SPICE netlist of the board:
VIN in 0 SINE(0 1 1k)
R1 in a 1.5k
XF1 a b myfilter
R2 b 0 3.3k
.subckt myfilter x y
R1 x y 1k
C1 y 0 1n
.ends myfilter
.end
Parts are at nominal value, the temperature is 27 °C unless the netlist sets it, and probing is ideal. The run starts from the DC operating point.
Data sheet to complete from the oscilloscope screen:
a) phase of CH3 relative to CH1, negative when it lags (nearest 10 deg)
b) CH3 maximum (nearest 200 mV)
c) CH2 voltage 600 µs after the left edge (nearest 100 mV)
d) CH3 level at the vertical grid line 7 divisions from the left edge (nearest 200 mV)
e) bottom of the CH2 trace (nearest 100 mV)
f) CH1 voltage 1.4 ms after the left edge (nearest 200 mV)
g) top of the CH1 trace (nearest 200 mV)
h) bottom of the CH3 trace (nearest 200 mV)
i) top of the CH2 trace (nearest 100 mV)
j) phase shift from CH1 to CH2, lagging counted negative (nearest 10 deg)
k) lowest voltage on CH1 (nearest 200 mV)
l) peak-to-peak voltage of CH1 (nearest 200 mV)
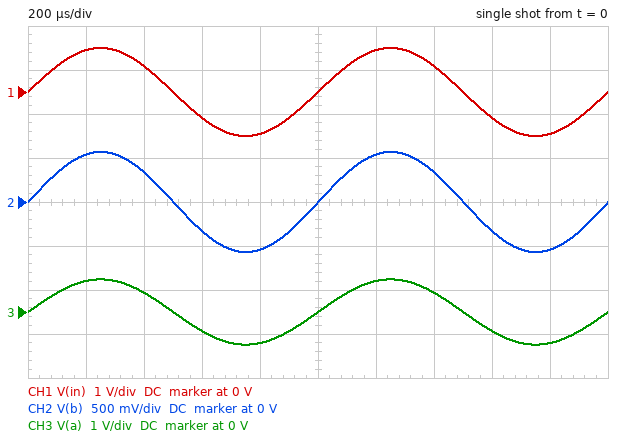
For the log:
0 deg
800 mV
-300 mV
400 mV
-600 mV
600 mV
1.0 V
-800 mV
600 mV
0 deg
-1.0 V
2.0 V
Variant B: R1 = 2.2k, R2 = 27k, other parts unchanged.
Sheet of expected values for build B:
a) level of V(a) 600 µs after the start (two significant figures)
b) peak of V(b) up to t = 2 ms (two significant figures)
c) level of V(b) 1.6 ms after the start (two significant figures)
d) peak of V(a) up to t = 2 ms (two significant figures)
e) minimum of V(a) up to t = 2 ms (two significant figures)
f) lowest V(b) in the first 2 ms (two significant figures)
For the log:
-540 mV
890 mV
-510 mV
930 mV
-930 mV
-890 mV
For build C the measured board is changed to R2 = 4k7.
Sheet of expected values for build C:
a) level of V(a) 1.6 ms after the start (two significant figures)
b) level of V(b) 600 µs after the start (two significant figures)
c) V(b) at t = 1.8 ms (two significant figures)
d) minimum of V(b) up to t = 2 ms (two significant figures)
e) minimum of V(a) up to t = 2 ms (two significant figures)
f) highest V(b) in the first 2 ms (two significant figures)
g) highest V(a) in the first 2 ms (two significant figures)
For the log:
-460 mV
-380 mV
-620 mV
-650 mV
-790 mV
650 mV
790 mV
